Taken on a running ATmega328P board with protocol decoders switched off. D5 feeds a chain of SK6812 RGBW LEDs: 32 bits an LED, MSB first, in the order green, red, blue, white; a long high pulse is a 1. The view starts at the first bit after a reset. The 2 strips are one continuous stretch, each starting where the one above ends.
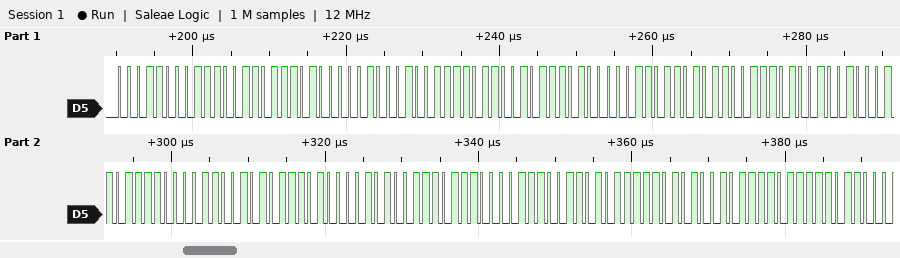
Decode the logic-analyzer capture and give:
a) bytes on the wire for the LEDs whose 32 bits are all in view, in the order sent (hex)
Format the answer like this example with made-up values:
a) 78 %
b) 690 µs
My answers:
a) 18 E6 E8 22 7B 2E 83 6B 3A 48 DE 19 5D 0A 77 0E 6B EA 5E FB
